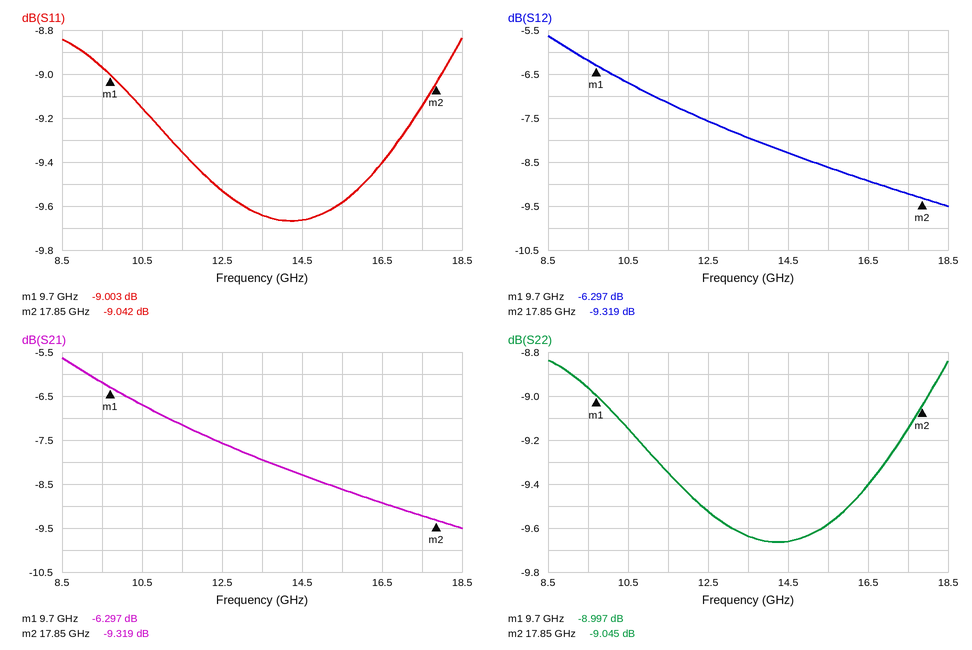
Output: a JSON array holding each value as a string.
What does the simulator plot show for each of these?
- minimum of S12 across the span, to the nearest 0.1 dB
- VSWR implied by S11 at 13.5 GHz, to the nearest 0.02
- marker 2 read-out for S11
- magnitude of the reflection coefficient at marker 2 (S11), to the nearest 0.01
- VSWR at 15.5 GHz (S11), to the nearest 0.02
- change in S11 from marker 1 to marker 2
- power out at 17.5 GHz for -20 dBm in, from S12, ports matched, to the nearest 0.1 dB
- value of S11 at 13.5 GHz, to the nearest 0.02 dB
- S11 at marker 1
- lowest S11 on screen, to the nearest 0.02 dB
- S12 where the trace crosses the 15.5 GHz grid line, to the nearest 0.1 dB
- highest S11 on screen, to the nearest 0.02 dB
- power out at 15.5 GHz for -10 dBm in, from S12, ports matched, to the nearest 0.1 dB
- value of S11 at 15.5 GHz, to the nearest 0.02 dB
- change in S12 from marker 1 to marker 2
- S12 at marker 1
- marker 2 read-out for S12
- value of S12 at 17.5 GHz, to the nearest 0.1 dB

["-9.5 dB", "1.98", "-9.042 dB", "0.35", "2.00", "-0.039 dB", "-29.2 dBm", "-9.64 dB", "-9.003 dB", "-9.66 dB", "-8.6 dB", "-8.84 dB", "-18.6 dBm", "-9.58 dB", "-3.022 dB", "-6.297 dB", "-9.319 dB", "-9.2 dB"]
